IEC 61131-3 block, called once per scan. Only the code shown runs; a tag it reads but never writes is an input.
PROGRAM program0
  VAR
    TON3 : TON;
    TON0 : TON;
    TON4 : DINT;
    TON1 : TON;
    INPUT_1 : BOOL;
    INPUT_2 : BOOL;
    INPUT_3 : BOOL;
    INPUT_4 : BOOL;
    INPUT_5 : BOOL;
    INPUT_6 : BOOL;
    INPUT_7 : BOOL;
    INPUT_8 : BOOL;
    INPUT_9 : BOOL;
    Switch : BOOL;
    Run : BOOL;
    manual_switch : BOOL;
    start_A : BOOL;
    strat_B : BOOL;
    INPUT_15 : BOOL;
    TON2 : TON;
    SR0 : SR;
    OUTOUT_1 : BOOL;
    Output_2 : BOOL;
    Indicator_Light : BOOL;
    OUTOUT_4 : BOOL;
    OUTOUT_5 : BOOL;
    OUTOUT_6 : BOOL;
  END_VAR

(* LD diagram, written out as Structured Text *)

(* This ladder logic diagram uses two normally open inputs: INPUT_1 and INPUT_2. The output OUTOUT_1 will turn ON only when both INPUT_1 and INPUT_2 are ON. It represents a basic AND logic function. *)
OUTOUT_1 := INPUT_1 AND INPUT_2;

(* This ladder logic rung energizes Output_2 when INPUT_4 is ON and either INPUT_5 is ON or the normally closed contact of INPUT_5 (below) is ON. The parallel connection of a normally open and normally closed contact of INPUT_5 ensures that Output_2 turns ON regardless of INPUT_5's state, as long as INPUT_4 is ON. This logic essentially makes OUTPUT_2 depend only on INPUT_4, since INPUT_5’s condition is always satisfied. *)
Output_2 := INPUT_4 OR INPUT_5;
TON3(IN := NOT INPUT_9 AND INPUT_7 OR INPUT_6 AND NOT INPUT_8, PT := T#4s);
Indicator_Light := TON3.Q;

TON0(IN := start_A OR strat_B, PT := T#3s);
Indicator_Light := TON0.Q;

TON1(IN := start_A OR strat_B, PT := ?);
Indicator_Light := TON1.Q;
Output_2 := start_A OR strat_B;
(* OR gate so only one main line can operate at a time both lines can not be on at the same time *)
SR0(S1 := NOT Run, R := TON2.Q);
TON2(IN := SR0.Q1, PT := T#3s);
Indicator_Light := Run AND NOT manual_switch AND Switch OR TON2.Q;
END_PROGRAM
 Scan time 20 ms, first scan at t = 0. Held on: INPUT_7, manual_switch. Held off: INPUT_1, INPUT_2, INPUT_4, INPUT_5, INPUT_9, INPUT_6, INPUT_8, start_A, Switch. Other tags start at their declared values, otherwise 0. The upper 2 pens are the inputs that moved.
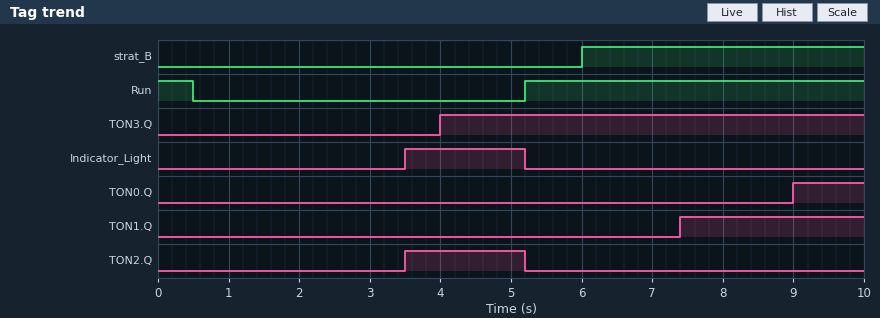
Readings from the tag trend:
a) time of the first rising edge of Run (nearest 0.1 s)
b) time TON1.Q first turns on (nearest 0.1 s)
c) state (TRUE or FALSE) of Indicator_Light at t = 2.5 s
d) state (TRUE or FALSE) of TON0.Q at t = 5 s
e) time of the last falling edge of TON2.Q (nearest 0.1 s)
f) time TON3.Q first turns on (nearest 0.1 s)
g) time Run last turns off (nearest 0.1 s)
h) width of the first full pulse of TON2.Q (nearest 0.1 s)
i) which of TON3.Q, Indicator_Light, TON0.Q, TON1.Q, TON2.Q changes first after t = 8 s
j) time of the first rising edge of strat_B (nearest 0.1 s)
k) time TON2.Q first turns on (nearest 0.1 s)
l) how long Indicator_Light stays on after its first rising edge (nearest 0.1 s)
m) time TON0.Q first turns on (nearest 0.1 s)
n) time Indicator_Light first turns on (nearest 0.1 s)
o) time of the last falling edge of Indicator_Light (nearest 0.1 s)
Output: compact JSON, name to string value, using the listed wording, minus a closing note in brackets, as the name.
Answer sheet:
{"time of the first rising edge of Run": "5.2 s", "time TON1.Q first turns on": "7.4 s", "state (TRUE or FALSE) of Indicator_Light at t = 2.5 s": "FALSE", "state (TRUE or FALSE) of TON0.Q at t = 5 s": "FALSE", "time of the last falling edge of TON2.Q": "5.2 s", "time TON3.Q first turns on": "4.0 s", "time Run last turns off": "0.5 s", "width of the first full pulse of TON2.Q": "1.7 s", "which of TON3.Q, Indicator_Light, TON0.Q, TON1.Q, TON2.Q changes first after t = 8 s": "TON0.Q", "time of the first rising edge of strat_B": "6.0 s", "time TON2.Q first turns on": "3.5 s", "how long Indicator_Light stays on after its first rising edge": "1.7 s", "time TON0.Q first turns on": "9.0 s", "time Indicator_Light first turns on": "3.5 s", "time of the last falling edge of Indicator_Light": "5.2 s"}
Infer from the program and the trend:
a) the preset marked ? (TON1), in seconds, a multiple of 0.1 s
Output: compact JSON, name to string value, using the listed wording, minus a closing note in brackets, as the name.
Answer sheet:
{"the preset marked ? (TON1), in seconds, a multiple of 0.1 s": "1.4 s"}
